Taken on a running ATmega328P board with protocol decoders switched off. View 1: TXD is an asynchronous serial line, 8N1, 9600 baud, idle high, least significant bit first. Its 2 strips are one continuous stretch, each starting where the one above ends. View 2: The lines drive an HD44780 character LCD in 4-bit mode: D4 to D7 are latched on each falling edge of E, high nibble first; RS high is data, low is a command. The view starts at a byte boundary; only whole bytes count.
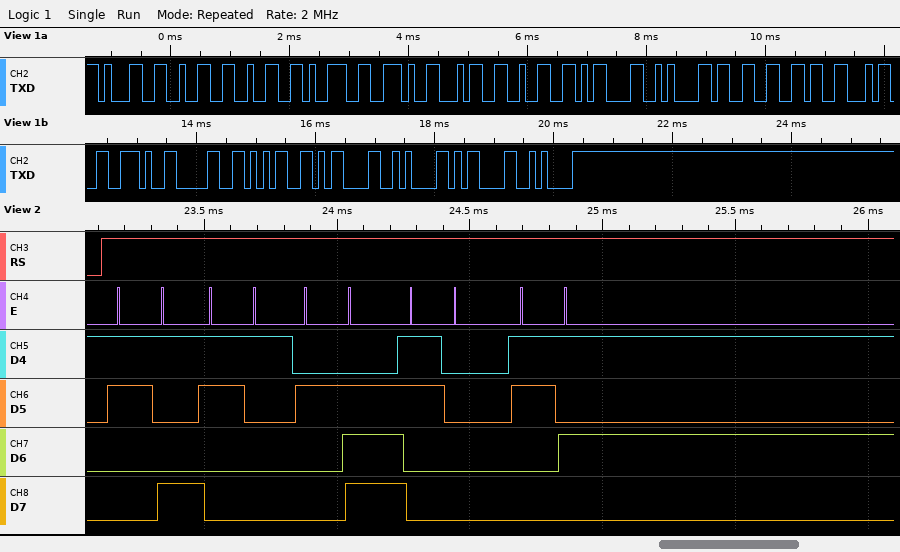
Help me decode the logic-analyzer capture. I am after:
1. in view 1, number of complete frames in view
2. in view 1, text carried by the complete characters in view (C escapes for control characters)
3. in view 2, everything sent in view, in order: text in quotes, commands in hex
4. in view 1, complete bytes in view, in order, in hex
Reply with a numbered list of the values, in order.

1. 19
2. "1229.42\r\n364.05\r\n\r\n"
3. "91.05"
4. 31 32 32 39 2E 34 32 0D 0A 33 36 34 2E 30 35 0D 0A 0D 0A
